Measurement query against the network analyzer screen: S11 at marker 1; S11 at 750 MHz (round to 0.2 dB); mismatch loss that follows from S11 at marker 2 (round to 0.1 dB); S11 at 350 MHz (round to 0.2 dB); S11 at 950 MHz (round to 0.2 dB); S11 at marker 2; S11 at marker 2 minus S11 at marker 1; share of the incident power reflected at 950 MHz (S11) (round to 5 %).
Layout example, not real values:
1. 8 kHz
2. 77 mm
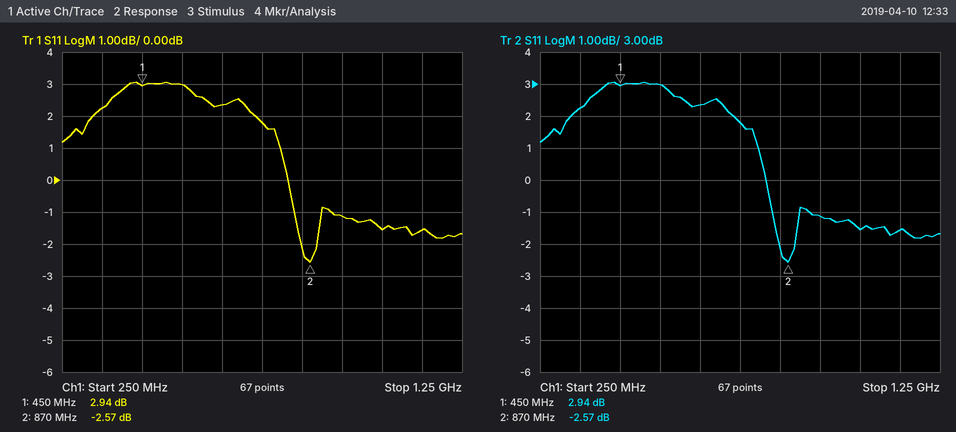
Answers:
1. 2.94 dB
2. 1.8 dB
3. 3.5 dB
4. 2.2 dB
5. -1.2 dB
6. -2.57 dB
7. -5.51 dB
8. 75 %
